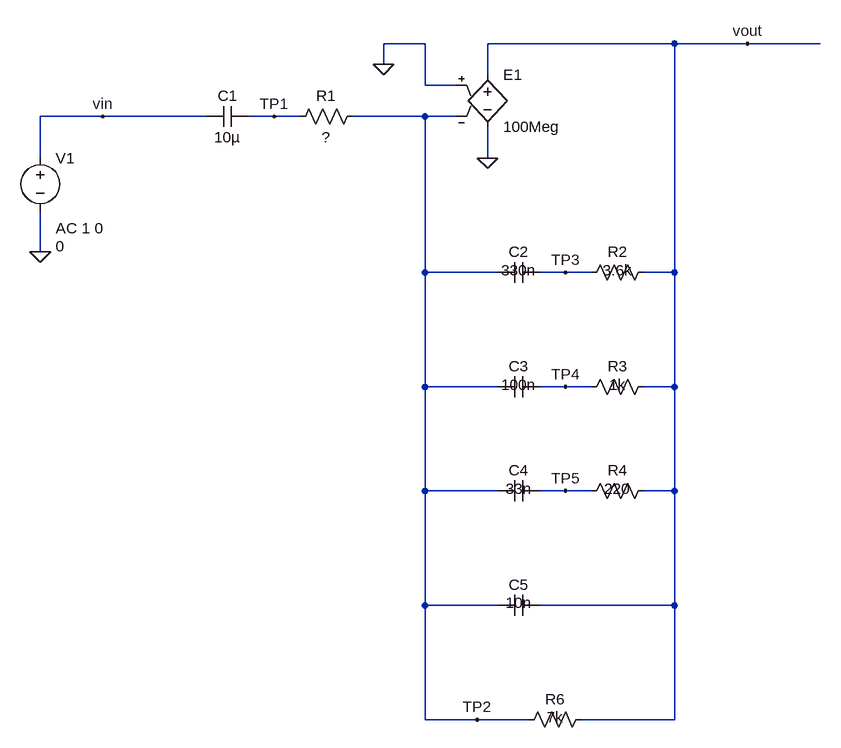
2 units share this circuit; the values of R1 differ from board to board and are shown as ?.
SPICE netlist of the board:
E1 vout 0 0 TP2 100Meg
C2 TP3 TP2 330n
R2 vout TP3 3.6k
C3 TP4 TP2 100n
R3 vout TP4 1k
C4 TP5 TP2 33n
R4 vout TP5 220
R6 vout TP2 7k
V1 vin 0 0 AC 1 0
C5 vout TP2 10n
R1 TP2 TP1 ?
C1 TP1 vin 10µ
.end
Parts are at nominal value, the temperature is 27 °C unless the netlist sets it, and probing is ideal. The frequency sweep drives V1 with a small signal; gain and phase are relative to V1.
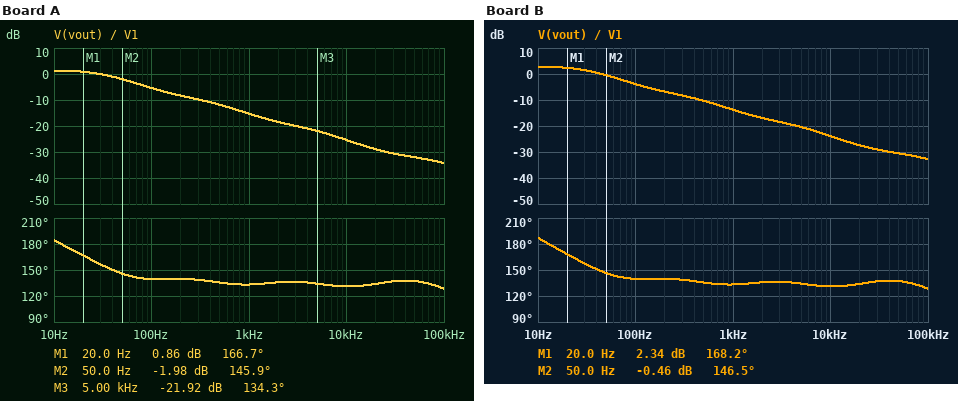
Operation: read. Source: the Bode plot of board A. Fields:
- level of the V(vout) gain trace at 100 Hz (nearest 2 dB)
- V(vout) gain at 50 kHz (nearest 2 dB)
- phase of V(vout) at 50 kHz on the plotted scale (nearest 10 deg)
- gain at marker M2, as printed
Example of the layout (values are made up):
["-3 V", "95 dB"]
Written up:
["-6 dB", "-32 dB", "140 deg", "-1.98 dB"]
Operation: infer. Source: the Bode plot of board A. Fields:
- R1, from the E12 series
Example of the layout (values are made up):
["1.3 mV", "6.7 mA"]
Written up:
["5.6 kΩ"]
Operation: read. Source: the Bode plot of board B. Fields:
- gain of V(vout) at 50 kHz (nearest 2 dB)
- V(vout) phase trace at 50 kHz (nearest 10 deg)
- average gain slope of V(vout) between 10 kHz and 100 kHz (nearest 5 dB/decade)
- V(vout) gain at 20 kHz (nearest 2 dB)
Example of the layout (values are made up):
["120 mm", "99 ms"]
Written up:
["-30 dB", "140 deg", "-10 dB/decade", "-28 dB"]
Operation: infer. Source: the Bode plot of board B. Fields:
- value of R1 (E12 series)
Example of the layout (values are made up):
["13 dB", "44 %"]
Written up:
["4.7 kΩ"]
